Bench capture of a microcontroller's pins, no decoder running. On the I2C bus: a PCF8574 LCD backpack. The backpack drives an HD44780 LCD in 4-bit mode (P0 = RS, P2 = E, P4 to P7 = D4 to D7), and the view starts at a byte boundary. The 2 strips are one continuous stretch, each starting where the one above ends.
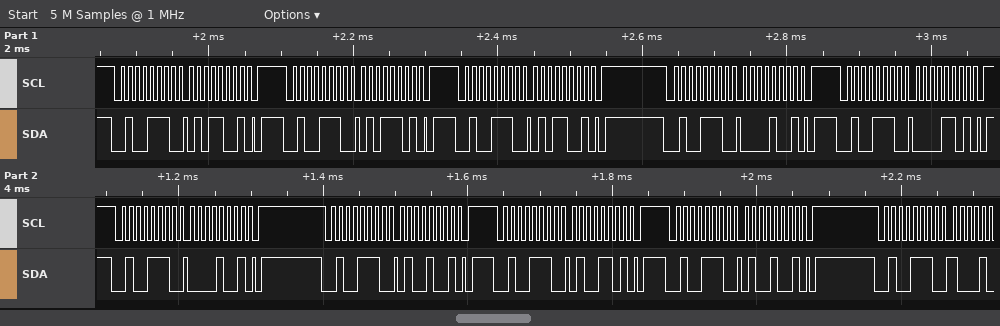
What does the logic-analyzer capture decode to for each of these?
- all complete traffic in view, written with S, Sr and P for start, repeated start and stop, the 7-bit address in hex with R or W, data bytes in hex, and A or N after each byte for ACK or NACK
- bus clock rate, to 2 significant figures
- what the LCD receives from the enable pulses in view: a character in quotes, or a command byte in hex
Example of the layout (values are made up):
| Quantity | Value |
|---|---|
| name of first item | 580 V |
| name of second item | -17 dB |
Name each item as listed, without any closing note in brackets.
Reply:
| Quantity | Value |
|---|---|
| all complete traffic in view, written with S, Sr and P for start, repeated start and stop, the 7-bit address in hex with R or W, data bytes in hex, and A or N after each byte for ACK or NACK | S 27W A 59 A P S 27W A 5D A P S 27W A 59 A P S 27W A 09 A P S 27W A 0D A P S 27W A 09 A P S 27W A 49 A P S 27W A 4D A P S 27W A 49 A P S 27W A |
| bus clock rate, to 2 significant figures | 100 kHz |
| what the LCD receives from the enable pulses in view: a character in quotes, or a command byte in hex | 'P' |
